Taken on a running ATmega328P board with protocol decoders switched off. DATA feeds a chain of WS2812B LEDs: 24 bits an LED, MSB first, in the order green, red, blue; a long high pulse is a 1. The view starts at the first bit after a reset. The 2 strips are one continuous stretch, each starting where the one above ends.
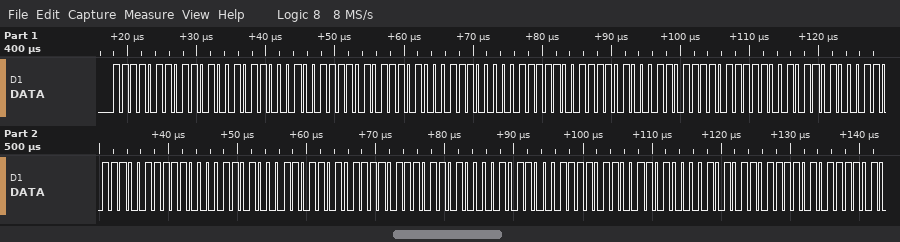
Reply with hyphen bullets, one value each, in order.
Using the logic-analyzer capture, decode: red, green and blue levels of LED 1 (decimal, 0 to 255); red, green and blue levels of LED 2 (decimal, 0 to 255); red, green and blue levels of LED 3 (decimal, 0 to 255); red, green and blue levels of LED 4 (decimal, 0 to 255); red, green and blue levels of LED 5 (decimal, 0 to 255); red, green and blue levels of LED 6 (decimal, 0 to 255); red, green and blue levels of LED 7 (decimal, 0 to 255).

- 210, 246, 196
- 209, 245, 193
- 209, 243, 189
- 209, 242, 185
- 209, 240, 181
- 208, 238, 177
- 208, 236, 173
